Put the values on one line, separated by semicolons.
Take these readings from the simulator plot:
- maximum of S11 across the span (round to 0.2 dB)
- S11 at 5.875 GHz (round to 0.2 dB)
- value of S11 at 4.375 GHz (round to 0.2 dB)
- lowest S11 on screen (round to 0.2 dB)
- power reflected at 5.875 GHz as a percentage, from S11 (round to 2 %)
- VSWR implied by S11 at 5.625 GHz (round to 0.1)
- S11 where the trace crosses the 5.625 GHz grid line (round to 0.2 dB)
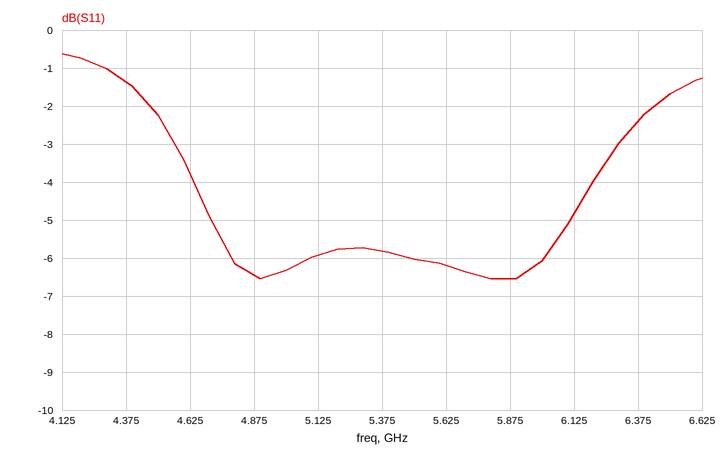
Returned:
-0.6 dB; -6.6 dB; -1.4 dB; -6.6 dB; 22 %; 2.9; -6.2 dB
